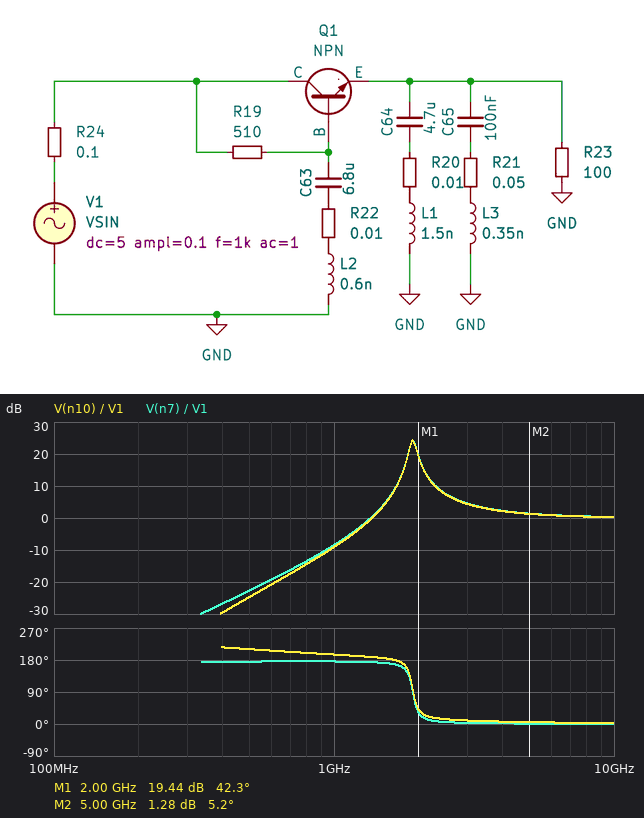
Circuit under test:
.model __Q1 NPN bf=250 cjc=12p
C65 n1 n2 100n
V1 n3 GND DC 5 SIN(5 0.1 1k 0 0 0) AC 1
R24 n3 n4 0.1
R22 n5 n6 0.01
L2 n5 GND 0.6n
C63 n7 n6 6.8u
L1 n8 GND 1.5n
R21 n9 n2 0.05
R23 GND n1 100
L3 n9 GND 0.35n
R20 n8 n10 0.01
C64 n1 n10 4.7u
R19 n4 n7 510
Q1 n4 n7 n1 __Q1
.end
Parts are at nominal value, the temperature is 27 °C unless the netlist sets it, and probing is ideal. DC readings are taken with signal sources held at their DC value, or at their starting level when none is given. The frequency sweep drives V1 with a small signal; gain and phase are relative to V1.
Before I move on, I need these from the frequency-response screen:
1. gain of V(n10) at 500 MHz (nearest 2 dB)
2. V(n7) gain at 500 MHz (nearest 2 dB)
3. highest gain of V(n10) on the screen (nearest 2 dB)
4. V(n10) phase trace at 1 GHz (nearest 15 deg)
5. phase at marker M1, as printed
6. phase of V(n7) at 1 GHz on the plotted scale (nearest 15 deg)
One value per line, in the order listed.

-24 dB
-22 dB
24 dB
195 deg
42.3 deg
180 deg
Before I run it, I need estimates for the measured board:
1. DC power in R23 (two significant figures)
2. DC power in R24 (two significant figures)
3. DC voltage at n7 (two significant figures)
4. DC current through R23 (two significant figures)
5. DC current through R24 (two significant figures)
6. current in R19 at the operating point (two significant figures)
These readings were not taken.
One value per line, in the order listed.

160 mW
160 µW
4.9 V
40 mA
40 mA
160 µA
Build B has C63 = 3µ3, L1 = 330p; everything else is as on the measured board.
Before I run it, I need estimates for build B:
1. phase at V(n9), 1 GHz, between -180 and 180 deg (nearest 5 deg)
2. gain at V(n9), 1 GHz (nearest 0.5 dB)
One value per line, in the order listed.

-155 deg
-10.0 dB
